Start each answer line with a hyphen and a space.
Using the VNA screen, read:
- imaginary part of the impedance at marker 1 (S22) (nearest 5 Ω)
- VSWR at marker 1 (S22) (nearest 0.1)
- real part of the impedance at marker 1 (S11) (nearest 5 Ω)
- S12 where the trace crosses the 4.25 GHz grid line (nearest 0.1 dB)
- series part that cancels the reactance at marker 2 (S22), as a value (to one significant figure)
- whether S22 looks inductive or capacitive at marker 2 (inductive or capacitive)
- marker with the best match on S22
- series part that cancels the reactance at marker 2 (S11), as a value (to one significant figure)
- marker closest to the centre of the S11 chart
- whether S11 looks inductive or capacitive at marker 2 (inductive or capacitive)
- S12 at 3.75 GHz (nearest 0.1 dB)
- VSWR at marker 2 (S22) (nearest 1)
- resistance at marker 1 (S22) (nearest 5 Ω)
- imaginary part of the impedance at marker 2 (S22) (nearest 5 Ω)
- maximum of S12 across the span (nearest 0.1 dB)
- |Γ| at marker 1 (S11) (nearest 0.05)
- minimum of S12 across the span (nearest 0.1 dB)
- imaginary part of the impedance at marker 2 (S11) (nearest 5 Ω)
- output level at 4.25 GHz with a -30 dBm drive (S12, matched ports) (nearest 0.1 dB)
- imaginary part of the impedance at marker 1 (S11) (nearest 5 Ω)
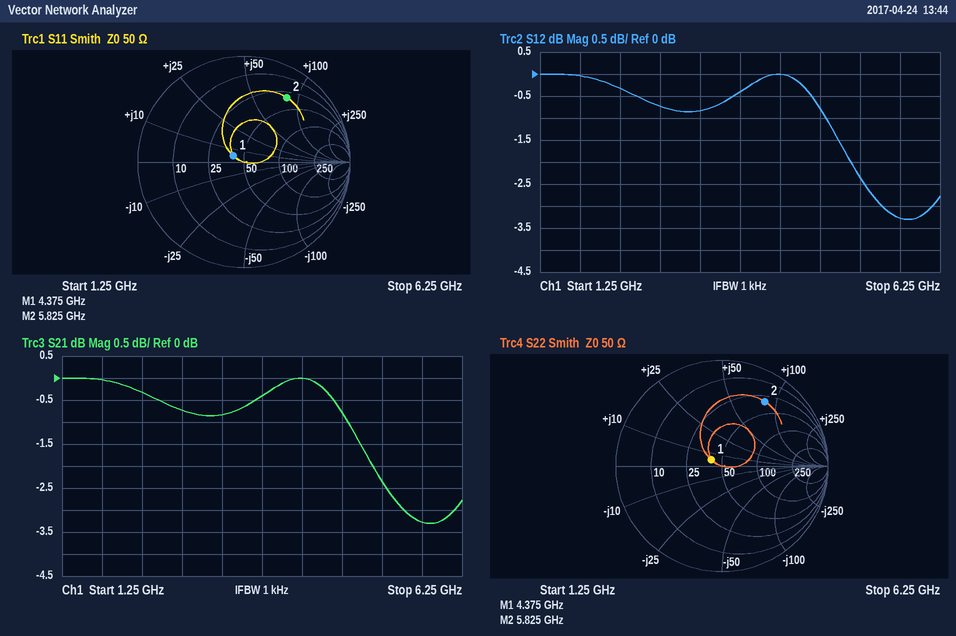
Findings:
- +5 Ω
- 1.3
- 40 Ω
- 0.0 dB
- 300 fF
- inductive
- marker 1
- 300 fF
- marker 1
- inductive
- -0.4 dB
- 6
- 40 Ω
- +85 Ω
- 0.0 dB
- 0.10
- -3.3 dB
- +85 Ω
- -30.0 dBm
- +5 Ω
